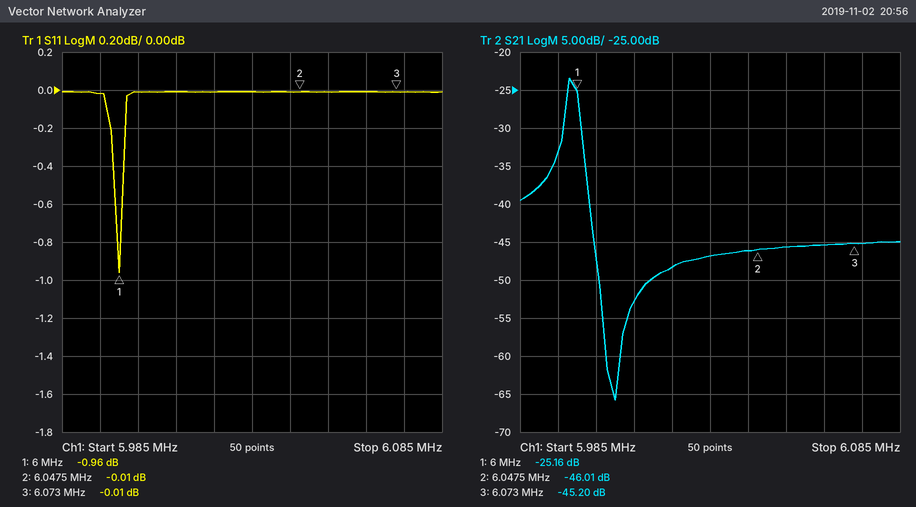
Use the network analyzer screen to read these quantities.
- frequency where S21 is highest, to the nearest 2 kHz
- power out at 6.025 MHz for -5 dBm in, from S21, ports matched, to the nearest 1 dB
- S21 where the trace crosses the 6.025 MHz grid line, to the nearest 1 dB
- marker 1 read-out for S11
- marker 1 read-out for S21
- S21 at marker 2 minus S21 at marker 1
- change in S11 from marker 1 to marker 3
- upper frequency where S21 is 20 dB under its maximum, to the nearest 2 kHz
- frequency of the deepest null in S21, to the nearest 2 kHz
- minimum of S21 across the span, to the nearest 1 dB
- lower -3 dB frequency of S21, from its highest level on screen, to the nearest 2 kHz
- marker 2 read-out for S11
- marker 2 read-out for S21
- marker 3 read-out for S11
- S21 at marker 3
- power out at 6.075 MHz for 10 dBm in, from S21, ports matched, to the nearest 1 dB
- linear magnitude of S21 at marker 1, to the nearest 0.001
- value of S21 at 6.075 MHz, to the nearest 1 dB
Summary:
5.998 MHz
-53 dBm
-48 dB
-0.96 dB
-25.16 dB
-20.85 dB
0.95 dB
6.004 MHz
6.010 MHz
-66 dB
5.998 MHz
-0.01 dB
-46.01 dB
-0.01 dB
-45.20 dB
-35 dBm
0.055
-45 dB
